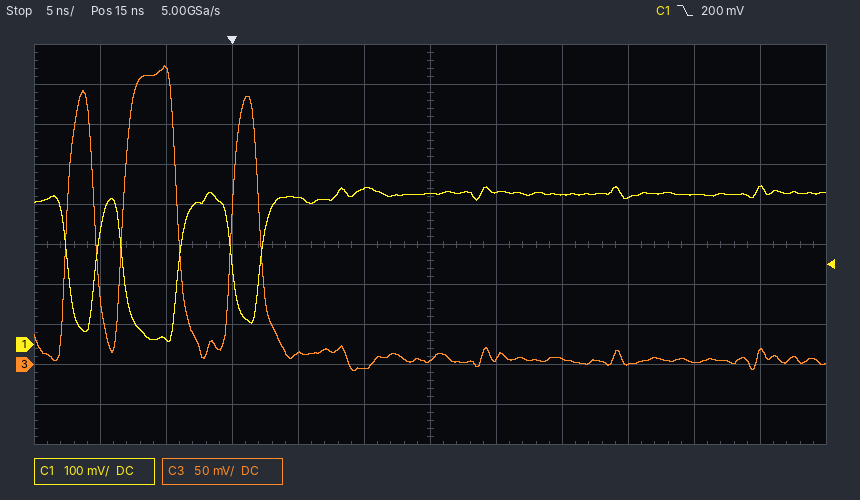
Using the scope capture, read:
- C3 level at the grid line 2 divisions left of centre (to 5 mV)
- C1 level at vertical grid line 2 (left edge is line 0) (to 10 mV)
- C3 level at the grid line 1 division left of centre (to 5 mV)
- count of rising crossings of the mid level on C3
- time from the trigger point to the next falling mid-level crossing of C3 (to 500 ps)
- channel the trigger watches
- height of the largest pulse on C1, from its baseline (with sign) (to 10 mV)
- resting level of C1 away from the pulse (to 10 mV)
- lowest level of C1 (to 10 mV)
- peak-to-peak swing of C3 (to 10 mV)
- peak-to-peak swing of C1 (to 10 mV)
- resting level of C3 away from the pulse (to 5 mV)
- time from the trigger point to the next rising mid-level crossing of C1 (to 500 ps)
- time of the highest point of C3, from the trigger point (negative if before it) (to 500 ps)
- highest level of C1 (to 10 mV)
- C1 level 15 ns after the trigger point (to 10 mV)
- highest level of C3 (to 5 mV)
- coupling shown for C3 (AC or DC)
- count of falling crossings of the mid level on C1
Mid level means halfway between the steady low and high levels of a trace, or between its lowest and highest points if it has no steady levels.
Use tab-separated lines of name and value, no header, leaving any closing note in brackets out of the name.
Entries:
C3 level at the grid line 2 divisions left of centre	15 mV
C1 level at vertical grid line 2 (left edge is line 0)	10 mV
C3 level at the grid line 1 division left of centre	-5 mV
count of rising crossings of the mid level on C3	3
time from the trigger point to the next falling mid-level crossing of C3	2.0 ns
channel the trigger watches	C1
height of the largest pulse on C1, from its baseline (with sign)	-370 mV
resting level of C1 away from the pulse	380 mV
lowest level of C1	10 mV
peak-to-peak swing of C3	380 mV
peak-to-peak swing of C1	390 mV
resting level of C3 away from the pulse	5 mV
time from the trigger point to the next rising mid-level crossing of C1	2.0 ns
time of the highest point of C3, from the trigger point (negative if before it)	-5.0 ns
highest level of C1	400 mV
C1 level 15 ns after the trigger point	380 mV
highest level of C3	375 mV
coupling shown for C3	DC
count of falling crossings of the mid level on C1	3
